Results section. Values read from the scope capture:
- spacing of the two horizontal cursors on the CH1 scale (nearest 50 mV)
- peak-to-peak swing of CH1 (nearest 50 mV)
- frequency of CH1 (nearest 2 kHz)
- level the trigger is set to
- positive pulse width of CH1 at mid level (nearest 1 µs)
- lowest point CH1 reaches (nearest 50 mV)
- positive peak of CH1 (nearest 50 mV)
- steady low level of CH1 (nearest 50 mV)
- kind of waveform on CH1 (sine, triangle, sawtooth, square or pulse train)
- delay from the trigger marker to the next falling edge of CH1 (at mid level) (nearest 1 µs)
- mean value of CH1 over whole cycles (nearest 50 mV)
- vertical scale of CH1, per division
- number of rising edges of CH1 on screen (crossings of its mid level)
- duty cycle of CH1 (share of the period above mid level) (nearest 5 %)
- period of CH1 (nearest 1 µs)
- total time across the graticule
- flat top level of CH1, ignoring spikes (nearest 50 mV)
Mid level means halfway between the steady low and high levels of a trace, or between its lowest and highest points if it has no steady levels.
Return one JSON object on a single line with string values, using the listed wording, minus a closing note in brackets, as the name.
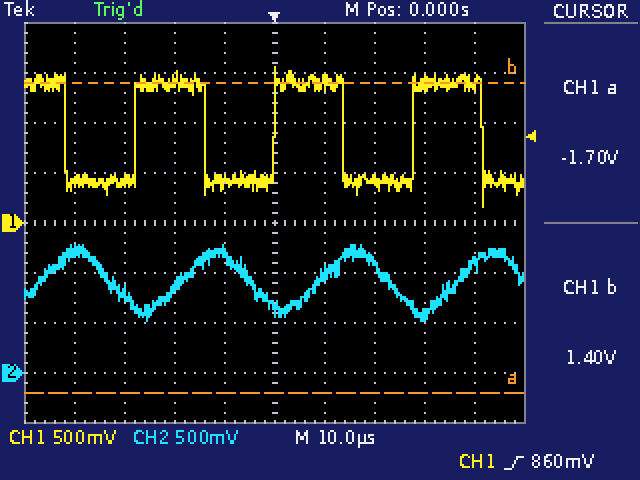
{"spacing of the two horizontal cursors on the CH1 scale": "3.10 V", "peak-to-peak swing of CH1": "1.40 V", "frequency of CH1": "36 kHz", "level the trigger is set to": "860 mV", "positive pulse width of CH1 at mid level": "14 µs", "lowest point CH1 reaches": "150 mV", "positive peak of CH1": "1.55 V", "steady low level of CH1": "400 mV", "kind of waveform on CH1": "square", "delay from the trigger marker to the next falling edge of CH1 (at mid level)": "14 µs", "mean value of CH1 over whole cycles": "900 mV", "vertical scale of CH1, per division": "500 mV", "number of rising edges of CH1 on screen": "3", "duty cycle of CH1 (share of the period above mid level)": "50 %", "period of CH1": "28 µs", "total time across the graticule": "100 µs", "flat top level of CH1, ignoring spikes": "1.40 V"}
